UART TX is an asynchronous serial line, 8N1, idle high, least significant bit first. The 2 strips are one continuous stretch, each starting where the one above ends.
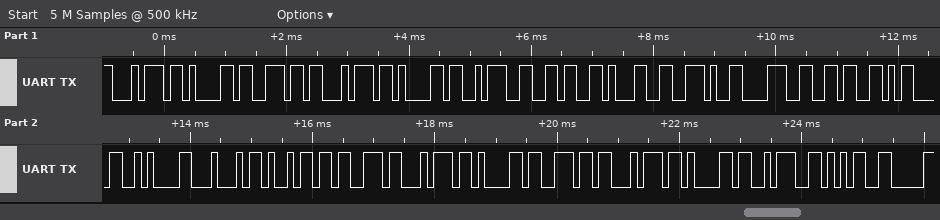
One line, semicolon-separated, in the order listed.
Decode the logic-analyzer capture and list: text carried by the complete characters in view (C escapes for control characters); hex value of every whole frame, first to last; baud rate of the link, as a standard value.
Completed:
"tanta:61.86\r\nDistanta:5"; 0x74 0x61 0x6E 0x74 0x61 0x3A 0x36 0x31 0x2E 0x38 0x36 0x0D 0x0A 0x44 0x69 0x73 0x74 0x61 0x6E 0x74 0x61 0x3A 0x35; 9600 baud
